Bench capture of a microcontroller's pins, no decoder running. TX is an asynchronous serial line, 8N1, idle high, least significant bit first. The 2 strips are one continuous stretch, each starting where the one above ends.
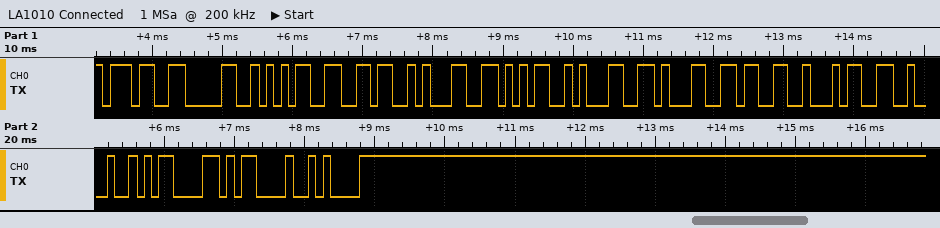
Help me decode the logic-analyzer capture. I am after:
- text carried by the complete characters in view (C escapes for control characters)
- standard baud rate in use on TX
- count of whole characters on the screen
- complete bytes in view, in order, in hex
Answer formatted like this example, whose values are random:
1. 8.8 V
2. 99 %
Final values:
1. "7056151134\"\r\r\n"
2. 9600 baud
3. 14
4. 0x37 0x30 0x35 0x36 0x31 0x35 0x31 0x31 0x33 0x34 0x22 0x0D 0x0D 0x0A
